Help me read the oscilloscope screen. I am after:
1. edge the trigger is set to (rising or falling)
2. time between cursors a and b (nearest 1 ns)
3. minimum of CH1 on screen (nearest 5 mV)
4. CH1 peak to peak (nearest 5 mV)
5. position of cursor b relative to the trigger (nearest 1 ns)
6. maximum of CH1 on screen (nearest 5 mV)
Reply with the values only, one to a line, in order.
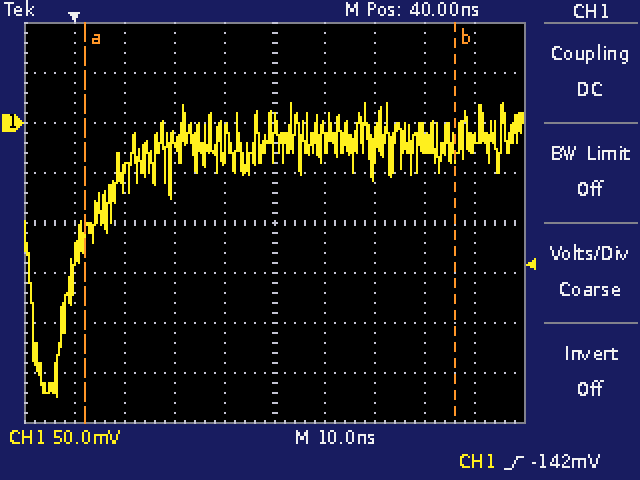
rising
74 ns
-275 mV
295 mV
+76 ns
20 mV
